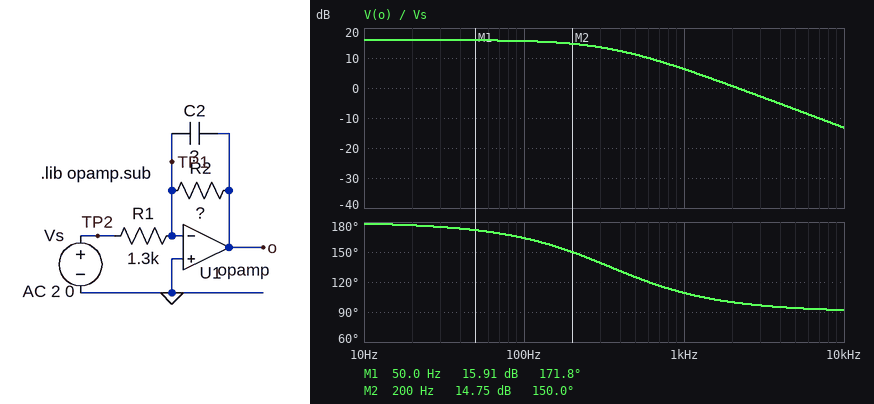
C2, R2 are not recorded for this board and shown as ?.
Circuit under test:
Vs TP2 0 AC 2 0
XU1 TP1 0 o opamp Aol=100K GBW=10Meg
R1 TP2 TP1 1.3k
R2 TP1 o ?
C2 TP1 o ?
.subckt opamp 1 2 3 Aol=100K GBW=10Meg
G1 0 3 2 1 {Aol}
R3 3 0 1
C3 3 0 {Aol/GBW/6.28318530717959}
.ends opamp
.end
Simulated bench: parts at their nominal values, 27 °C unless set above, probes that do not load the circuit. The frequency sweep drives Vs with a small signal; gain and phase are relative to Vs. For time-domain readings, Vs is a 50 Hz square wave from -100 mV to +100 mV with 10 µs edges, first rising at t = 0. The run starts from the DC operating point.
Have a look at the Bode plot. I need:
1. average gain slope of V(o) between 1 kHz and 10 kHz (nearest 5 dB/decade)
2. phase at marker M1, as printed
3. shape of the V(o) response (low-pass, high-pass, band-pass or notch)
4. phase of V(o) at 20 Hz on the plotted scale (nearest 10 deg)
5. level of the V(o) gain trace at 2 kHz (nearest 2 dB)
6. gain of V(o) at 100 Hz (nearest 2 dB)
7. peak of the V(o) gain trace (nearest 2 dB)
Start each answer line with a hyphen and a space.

- -20 dB/decade
- 171.8 deg
- low-pass
- 180 deg
- 0 dB
- 16 dB
- 16 dB
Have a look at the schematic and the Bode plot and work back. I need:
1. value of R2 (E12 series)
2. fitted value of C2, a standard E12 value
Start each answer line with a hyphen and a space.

- 8.2 kΩ
- 56 nF
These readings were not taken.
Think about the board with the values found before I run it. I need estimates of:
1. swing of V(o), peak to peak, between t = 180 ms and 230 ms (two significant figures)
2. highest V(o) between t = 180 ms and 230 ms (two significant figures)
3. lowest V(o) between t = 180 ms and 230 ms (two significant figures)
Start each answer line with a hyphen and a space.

- 1.3 V
- 630 mV
- -630 mV
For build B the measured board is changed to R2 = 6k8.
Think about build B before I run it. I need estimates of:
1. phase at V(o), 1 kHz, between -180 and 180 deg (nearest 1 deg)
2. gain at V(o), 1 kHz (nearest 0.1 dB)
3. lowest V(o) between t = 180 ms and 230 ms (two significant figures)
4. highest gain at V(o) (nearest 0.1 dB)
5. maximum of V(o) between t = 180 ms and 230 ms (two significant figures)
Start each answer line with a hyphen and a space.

- 113 deg
- 6.1 dB
- -520 mV
- 14.4 dB
- 520 mV
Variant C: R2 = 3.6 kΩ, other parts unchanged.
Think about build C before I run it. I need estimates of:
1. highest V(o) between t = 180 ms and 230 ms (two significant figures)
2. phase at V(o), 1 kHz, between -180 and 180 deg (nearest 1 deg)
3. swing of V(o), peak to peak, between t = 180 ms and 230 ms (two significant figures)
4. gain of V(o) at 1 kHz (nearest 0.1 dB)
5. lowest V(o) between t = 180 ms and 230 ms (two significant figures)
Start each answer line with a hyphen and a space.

- 280 mV
- 128 deg
- 550 mV
- 4.7 dB
- -280 mV
